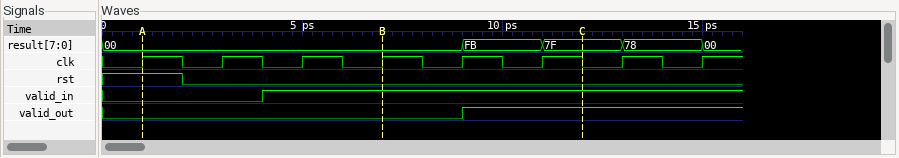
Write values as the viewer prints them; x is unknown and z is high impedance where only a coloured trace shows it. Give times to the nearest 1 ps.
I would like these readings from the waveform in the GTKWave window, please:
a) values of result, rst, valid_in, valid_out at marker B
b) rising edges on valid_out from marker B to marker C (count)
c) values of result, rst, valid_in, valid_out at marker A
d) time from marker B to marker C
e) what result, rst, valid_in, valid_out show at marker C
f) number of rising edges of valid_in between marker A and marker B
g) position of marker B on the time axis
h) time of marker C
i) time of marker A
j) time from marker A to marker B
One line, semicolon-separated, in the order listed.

result=00, rst=0, valid_in=1, valid_out=0; 1; result=00, rst=1, valid_in=0, valid_out=0; 5 ps; result=7F, rst=0, valid_in=1, valid_out=1; 1; 7 ps; 12 ps; 1 ps; 6 ps
